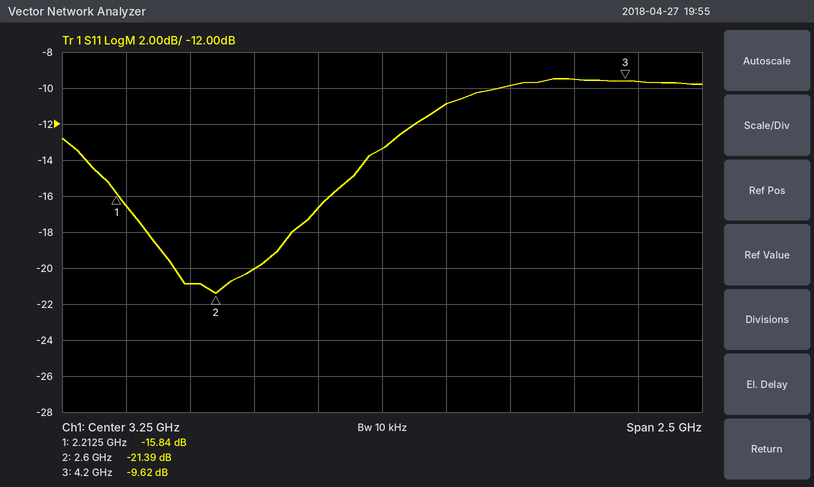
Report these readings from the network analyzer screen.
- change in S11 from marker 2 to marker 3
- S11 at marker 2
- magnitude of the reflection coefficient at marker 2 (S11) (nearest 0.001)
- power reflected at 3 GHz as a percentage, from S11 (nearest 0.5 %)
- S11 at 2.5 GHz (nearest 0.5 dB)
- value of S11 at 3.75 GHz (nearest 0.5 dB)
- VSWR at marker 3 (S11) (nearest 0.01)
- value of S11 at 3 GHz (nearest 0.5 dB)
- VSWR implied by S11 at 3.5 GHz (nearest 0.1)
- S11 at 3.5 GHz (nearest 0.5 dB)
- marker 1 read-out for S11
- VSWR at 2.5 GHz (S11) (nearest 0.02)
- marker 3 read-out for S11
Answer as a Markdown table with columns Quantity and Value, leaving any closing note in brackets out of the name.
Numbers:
| Quantity | Value |
|---|---|
| change in S11 from marker 2 to marker 3 | 11.77 dB |
| S11 at marker 2 | -21.39 dB |
| magnitude of the reflection coefficient at marker 2 (S11) | 0.085 |
| power reflected at 3 GHz as a percentage, from S11 | 2.0 % |
| S11 at 2.5 GHz | -21.0 dB |
| value of S11 at 3.75 GHz | -10.0 dB |
| VSWR at marker 3 (S11) | 1.99 |
| value of S11 at 3 GHz | -16.5 dB |
| VSWR implied by S11 at 3.5 GHz | 1.8 |
| S11 at 3.5 GHz | -11.0 dB |
| marker 1 read-out for S11 | -15.84 dB |
| VSWR at 2.5 GHz (S11) | 1.20 |
| marker 3 read-out for S11 | -9.62 dB |
